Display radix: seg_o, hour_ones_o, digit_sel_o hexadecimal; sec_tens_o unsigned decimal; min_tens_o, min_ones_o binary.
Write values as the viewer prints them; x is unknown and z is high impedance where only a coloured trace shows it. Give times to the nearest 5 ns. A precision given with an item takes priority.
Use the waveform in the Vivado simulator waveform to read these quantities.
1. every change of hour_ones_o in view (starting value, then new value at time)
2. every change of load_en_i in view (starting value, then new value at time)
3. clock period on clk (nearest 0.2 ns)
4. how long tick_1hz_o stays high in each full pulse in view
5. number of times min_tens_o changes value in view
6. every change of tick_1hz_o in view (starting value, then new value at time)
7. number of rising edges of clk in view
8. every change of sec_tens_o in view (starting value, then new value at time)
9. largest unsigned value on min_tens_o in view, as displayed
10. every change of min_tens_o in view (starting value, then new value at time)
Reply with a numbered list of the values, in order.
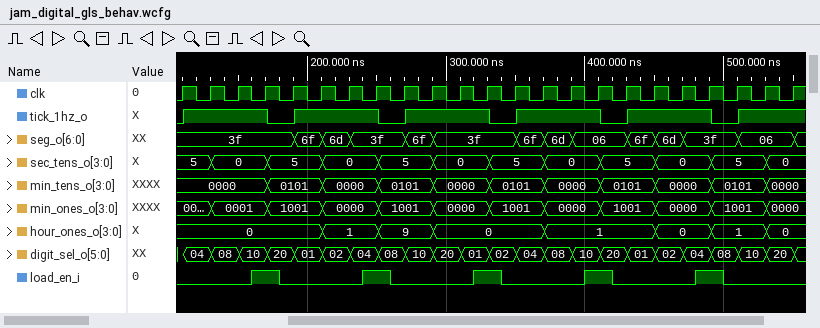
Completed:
1. 0, 1 at 210 ns, 9 at 250 ns, 0 at 290 ns, 1 at 370 ns, 0 at 450 ns, 1 at 490 ns, 0 at 530 ns
2. 0, 1 at 160 ns, 0 at 180 ns, 1 at 240 ns, 0 at 260 ns, 1 at 320 ns, 0 at 340 ns, 1 at 400 ns, 0 at 420 ns, 1 at 480 ns, 0 at 500 ns
3. 20 ns
4. 60 ns, 60 ns, 60 ns, 60 ns, 60 ns
5. 10
6. 0, 1 at 110 ns, 0 at 170 ns, 1 at 190 ns, 0 at 250 ns, 1 at 270 ns, 0 at 330 ns, 1 at 350 ns, 0 at 410 ns, 1 at 430 ns, 0 at 490 ns, 1 at 510 ns
7. 23
8. 5, 0 at 130 ns, 5 at 170 ns, 0 at 210 ns, 5 at 250 ns, 0 at 290 ns, 5 at 330 ns, 0 at 370 ns, 5 at 410 ns, 0 at 450 ns, 5 at 490 ns, 0 at 530 ns
9. 0101
10. 0000, 0101 at 170 ns, 0000 at 210 ns, 0101 at 250 ns, 0000 at 290 ns, 0101 at 330 ns, 0000 at 370 ns, 0101 at 410 ns, 0000 at 450 ns, 0101 at 490 ns, 0000 at 530 ns
